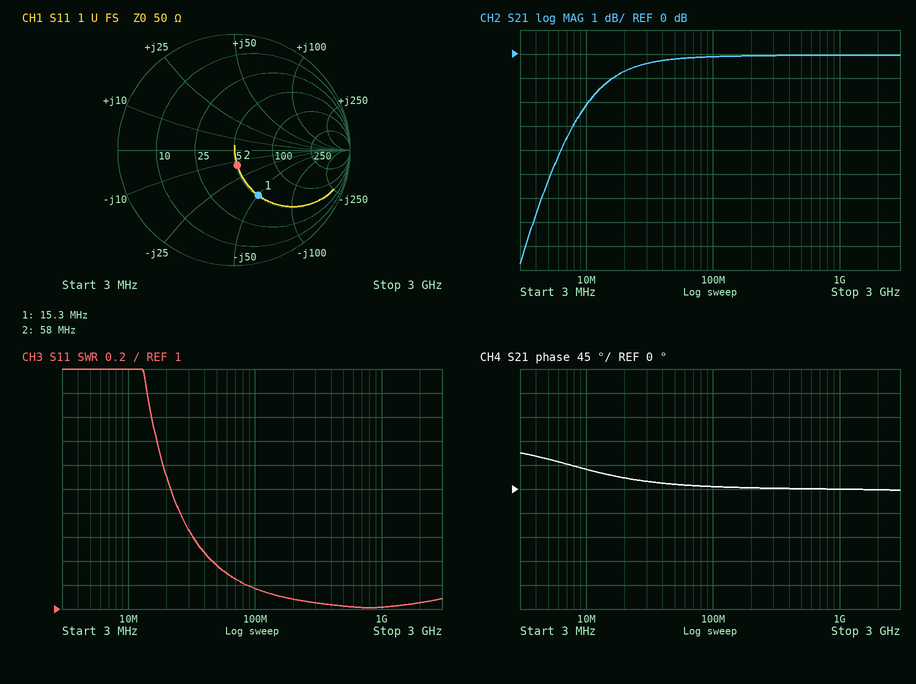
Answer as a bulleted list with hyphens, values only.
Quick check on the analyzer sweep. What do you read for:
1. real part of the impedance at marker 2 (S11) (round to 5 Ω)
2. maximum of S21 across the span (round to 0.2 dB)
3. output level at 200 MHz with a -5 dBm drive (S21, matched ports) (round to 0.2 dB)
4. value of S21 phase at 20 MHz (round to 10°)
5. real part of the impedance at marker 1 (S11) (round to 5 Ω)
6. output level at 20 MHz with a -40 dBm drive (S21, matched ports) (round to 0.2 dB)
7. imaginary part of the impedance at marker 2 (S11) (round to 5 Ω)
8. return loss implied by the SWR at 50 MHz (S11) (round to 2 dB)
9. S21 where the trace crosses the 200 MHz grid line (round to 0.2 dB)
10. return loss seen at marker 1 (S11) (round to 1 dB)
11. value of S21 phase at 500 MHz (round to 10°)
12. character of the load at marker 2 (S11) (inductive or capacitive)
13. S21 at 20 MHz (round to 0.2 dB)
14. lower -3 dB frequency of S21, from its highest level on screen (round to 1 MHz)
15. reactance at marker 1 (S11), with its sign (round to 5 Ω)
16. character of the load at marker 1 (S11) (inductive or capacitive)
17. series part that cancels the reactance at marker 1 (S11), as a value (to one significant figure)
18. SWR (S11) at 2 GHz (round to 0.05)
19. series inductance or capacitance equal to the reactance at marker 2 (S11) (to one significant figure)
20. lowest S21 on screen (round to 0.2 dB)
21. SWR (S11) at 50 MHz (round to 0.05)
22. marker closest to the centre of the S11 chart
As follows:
- 50 Ω
- 0.0 dB
- -5.0 dBm
- 20°
- 50 Ω
- -40.8 dBm
- -15 Ω
- 16 dB
- 0.0 dB
- 7 dB
- 0°
- capacitive
- -0.8 dB
- 8 MHz
- -50 Ω
- capacitive
- 500 nH
- 1.05
- 200 pF
- -8.8 dB
- 1.35
- marker 2
